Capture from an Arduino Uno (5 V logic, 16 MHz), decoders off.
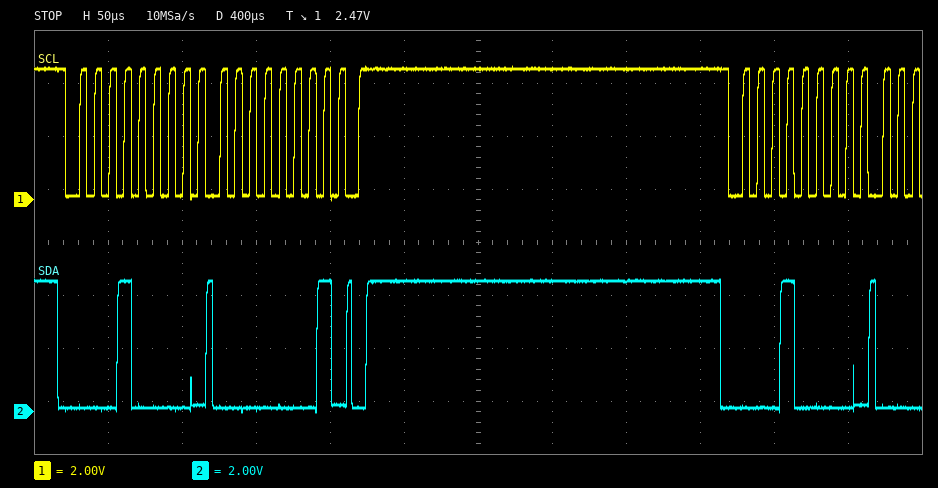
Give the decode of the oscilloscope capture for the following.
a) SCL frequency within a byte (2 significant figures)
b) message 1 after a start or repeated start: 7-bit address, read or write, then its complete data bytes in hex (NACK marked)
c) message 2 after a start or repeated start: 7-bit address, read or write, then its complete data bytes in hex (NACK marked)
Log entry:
100 kHz
0x08 write: 01
0x08 write
